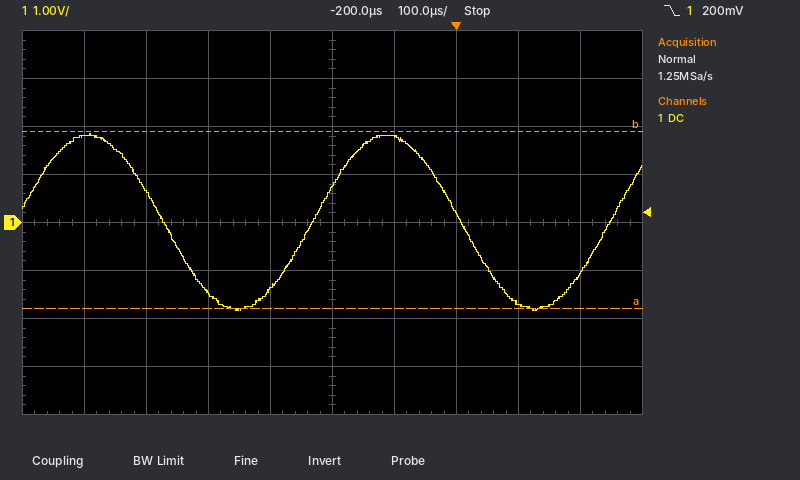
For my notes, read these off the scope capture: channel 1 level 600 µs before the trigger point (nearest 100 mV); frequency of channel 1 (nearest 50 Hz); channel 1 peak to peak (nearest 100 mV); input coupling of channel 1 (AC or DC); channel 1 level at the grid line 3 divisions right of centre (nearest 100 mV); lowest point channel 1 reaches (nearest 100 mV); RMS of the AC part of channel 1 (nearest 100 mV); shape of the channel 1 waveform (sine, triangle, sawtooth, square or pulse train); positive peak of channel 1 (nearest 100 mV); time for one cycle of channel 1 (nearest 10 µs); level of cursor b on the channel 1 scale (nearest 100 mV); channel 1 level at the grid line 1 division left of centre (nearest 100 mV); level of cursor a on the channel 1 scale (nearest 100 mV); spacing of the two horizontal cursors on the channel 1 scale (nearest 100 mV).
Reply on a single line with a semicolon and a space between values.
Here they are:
1.8 V; 2.10 kHz; 3.7 V; DC; -1.7 V; -1.8 V; 1.3 V; sine; 1.9 V; 480 µs; 1.9 V; -1.4 V; -1.8 V; 3.7 V
